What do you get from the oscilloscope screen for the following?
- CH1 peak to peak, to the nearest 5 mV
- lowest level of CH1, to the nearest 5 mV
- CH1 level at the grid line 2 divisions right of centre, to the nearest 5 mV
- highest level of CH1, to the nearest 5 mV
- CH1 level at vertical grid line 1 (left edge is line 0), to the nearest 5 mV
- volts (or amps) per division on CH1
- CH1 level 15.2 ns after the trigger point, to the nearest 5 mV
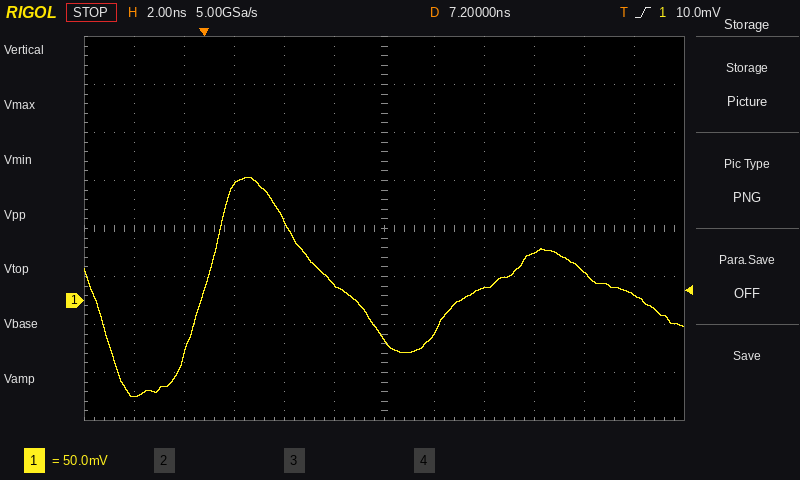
230 mV
-100 mV
15 mV
130 mV
-100 mV
50 mV
30 mV
